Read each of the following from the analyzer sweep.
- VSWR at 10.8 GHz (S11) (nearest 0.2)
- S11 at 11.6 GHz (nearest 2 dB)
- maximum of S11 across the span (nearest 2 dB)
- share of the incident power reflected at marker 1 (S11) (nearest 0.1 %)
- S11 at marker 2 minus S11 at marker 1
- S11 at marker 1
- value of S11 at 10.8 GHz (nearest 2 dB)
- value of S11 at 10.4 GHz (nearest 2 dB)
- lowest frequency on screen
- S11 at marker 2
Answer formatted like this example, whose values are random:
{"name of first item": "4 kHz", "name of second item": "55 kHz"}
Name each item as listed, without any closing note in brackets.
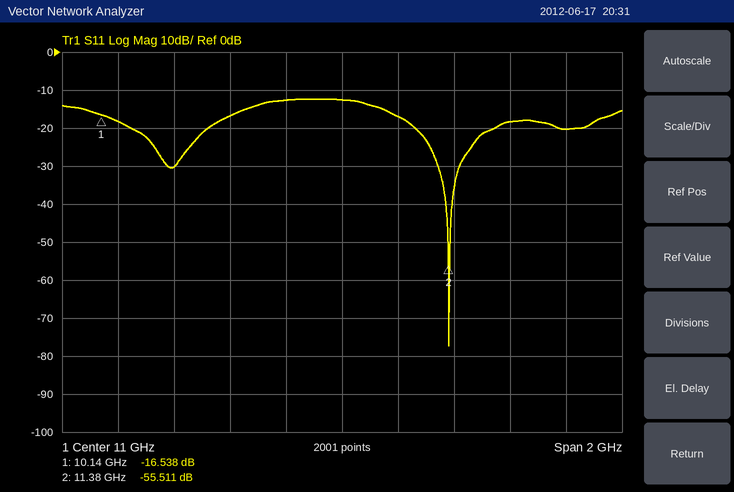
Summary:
{"VSWR at 10.8 GHz (S11)": "1.6", "S11 at 11.6 GHz": "-18 dB", "maximum of S11 across the span": "-12 dB", "share of the incident power reflected at marker 1 (S11)": "2.2 %", "S11 at marker 2 minus S11 at marker 1": "-38.973 dB", "S11 at marker 1": "-16.538 dB", "value of S11 at 10.8 GHz": "-12 dB", "value of S11 at 10.4 GHz": "-30 dB", "lowest frequency on screen": "10 GHz", "S11 at marker 2": "-55.511 dB"}
